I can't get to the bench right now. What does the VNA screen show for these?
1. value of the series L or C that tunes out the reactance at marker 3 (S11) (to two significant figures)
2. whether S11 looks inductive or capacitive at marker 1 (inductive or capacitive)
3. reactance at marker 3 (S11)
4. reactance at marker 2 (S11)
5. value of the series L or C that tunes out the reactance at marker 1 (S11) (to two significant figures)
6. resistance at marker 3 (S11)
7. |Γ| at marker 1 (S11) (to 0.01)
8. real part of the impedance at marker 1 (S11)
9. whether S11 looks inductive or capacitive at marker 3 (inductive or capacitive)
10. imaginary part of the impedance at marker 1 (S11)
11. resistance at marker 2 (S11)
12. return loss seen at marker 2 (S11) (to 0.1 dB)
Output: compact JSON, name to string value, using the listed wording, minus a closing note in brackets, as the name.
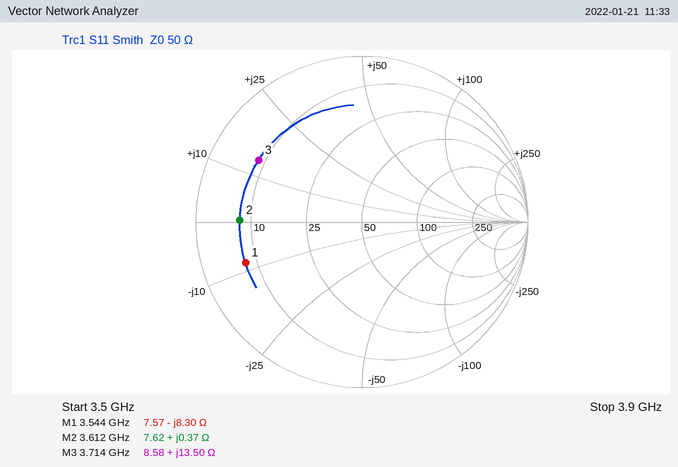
{"value of the series L or C that tunes out the reactance at marker 3 (S11)": "3.2 pF", "whether S11 looks inductive or capacitive at marker 1": "capacitive", "reactance at marker 3": "+13.50 Ω", "reactance at marker 2": "+0.37 Ω", "value of the series L or C that tunes out the reactance at marker 1 (S11)": "370 pH", "resistance at marker 3": "8.58 Ω", "|Γ| at marker 1 (S11)": "0.74", "real part of the impedance at marker 1": "7.57 Ω", "whether S11 looks inductive or capacitive at marker 3": "inductive", "imaginary part of the impedance at marker 1": "-8.30 Ω", "resistance at marker 2": "7.62 Ω", "return loss seen at marker 2 (S11)": "2.7 dB"}
